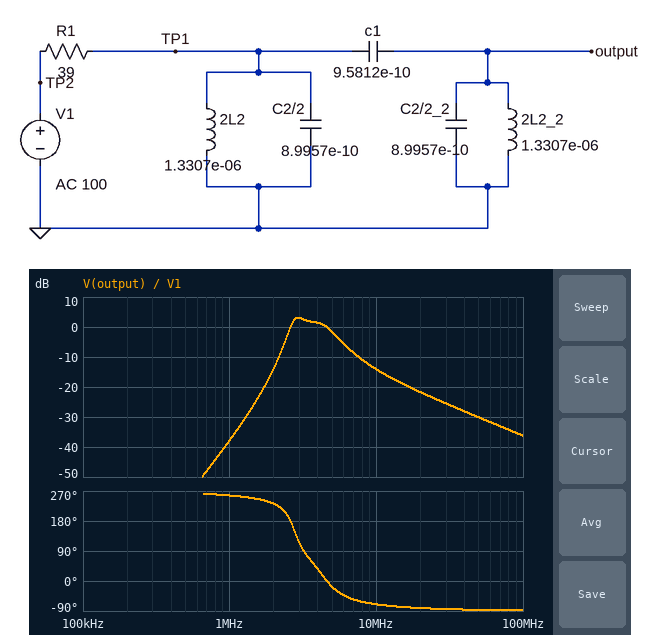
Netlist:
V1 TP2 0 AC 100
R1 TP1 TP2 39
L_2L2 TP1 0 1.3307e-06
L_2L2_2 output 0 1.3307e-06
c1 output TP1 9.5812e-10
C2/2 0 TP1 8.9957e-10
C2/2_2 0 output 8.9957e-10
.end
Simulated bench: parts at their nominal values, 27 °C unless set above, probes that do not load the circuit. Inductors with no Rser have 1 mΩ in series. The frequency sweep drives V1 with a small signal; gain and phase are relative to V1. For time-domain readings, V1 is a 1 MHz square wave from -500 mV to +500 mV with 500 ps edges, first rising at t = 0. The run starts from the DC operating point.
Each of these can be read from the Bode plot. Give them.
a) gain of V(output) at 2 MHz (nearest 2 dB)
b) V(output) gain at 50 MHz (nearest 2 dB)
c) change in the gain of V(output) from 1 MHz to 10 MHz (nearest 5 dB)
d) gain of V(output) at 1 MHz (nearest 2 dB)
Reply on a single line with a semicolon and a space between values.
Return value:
-14 dB; -30 dB; 25 dB; -38 dB
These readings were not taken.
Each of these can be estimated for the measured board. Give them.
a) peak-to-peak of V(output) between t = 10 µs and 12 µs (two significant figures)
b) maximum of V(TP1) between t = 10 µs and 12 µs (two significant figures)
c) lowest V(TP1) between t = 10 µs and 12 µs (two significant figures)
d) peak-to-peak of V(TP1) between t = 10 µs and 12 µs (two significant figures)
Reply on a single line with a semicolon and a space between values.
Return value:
830 mV; 330 mV; -330 mV; 660 mV
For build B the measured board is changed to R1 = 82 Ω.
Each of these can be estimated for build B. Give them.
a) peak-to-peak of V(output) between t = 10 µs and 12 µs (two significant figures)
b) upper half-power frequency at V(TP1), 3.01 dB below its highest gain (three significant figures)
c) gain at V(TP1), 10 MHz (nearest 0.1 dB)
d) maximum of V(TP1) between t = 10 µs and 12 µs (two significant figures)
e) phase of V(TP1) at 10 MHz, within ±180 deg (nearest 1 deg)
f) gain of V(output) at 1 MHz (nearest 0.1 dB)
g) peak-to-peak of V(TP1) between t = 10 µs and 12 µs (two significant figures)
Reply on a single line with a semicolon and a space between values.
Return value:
490 mV; 5.23 MHz; -15.3 dB; 200 mV; -80 deg; -44.0 dB; 400 mV
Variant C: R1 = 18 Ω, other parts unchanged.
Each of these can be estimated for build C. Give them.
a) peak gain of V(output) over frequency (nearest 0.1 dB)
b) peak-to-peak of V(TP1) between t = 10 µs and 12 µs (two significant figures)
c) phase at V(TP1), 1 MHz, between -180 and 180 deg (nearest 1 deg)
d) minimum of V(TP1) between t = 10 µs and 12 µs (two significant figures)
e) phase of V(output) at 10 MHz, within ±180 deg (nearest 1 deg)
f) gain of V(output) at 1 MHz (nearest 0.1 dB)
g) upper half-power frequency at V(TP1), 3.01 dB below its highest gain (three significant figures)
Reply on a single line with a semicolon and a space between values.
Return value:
9.2 dB; 1.1 V; 63 deg; -540 mV; -52 deg; -31.8 dB; 8.61 MHz
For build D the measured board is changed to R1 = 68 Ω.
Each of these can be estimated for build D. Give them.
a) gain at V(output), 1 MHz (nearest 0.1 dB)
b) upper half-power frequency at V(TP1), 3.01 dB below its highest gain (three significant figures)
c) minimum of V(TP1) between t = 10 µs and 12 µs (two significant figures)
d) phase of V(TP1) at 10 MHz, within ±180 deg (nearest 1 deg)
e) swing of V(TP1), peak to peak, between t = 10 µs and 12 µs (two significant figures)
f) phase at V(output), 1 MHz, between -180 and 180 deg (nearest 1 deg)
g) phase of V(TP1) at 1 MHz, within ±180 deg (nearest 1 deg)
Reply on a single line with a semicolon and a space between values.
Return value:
-42.4 dB; 5.38 MHz; -230 mV; -78 deg; 450 mV; -98 deg; 82 deg
